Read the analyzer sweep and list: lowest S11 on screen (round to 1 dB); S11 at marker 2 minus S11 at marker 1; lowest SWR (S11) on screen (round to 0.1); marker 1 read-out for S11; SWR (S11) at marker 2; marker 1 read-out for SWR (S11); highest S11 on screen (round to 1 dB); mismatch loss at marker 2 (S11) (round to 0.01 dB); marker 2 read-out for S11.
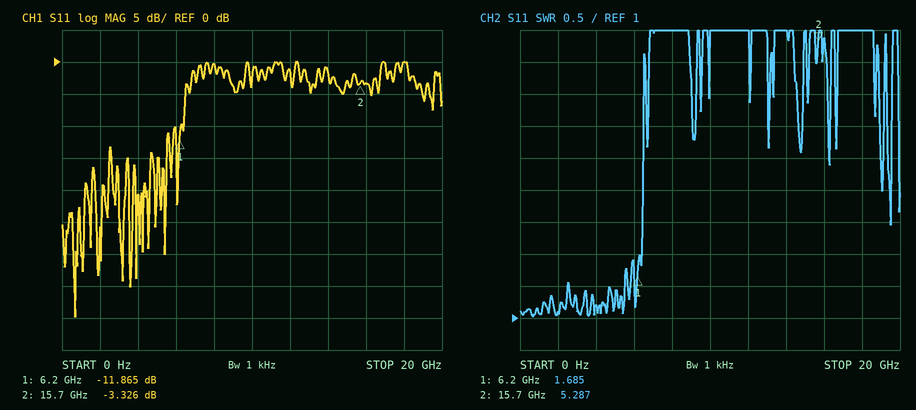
-40 dB
8.539 dB
1.0
-11.865 dB
5.287
1.685
0 dB
2.72 dB
-3.326 dB
